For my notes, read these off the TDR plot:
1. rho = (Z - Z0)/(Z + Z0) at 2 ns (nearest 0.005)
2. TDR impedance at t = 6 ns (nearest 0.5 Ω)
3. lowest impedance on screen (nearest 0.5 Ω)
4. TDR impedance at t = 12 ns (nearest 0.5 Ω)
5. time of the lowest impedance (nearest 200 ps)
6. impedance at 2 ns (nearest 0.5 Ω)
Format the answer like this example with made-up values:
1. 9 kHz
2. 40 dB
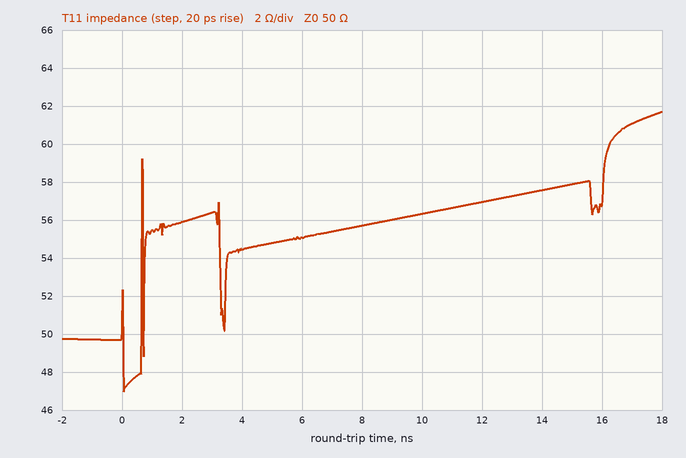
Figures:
1. +0.055
2. 55.0 Ω
3. 47.0 Ω
4. 57.0 Ω
5. 0.0 ns
6. 56.0 Ω
